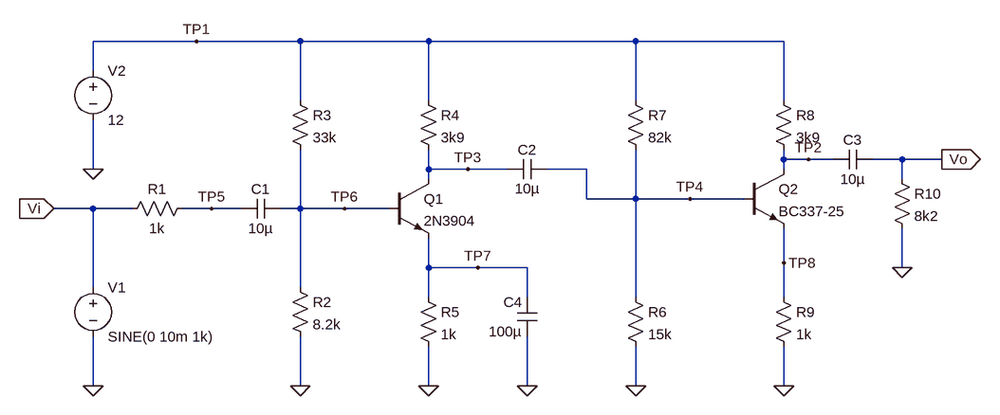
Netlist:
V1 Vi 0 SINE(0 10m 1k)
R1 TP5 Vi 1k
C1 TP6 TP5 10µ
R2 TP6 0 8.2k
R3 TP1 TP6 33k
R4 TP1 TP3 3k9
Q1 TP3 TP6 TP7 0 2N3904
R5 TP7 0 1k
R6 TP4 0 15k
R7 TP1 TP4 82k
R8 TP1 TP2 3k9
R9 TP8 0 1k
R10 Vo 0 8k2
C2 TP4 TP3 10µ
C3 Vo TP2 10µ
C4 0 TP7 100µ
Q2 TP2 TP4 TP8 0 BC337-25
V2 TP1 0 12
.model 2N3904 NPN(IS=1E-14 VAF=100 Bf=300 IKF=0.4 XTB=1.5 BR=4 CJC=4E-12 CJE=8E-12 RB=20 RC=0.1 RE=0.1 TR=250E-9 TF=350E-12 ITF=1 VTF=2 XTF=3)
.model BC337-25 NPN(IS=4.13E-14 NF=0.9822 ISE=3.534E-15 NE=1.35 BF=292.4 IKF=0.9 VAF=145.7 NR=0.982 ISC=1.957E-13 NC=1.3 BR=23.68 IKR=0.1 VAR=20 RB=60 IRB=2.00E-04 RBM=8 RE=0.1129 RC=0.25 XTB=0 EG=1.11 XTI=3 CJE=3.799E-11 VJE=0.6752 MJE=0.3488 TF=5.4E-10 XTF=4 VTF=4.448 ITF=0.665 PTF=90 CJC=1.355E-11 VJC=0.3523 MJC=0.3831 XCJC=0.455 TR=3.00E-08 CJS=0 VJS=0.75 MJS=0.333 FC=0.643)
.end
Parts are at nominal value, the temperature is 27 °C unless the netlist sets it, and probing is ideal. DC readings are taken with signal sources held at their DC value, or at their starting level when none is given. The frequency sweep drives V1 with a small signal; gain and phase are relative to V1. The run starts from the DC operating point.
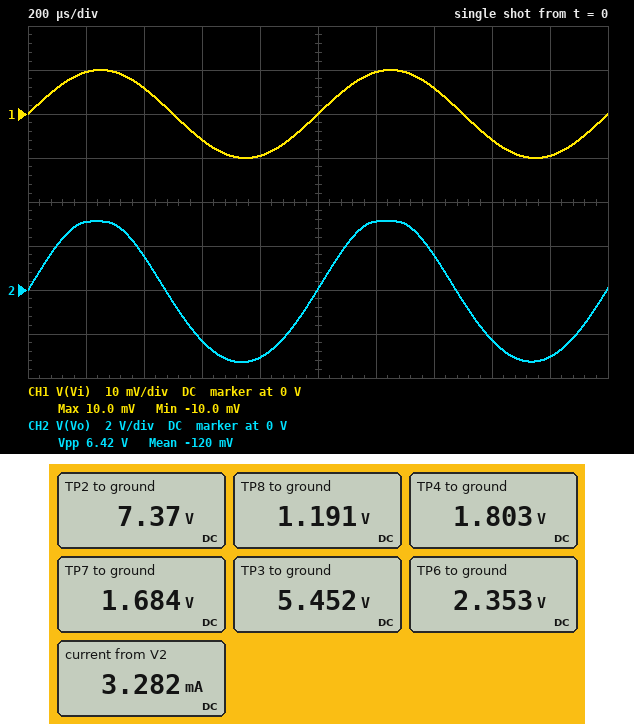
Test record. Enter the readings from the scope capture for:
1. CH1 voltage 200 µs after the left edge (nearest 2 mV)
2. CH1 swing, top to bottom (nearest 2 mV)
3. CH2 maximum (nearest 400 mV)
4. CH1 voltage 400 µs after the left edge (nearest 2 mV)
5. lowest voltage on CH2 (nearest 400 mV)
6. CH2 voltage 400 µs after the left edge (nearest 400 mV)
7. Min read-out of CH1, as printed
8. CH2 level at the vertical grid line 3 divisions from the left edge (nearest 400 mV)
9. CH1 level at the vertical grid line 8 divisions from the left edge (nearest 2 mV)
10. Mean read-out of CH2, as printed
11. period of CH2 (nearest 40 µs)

10 mV
20 mV
3.2 V
6 mV
-3.2 V
1.6 V
-10.0 mV
-2.4 V
-6 mV
-120 mV
1.00 ms
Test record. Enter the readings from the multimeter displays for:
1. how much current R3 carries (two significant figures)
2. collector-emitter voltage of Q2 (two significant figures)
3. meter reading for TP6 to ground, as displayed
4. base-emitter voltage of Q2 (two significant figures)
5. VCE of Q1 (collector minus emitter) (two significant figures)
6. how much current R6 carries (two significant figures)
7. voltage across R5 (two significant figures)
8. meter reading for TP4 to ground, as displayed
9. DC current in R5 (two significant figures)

290 µA
6.2 V
2.353 V
610 mV
3.8 V
120 µA
1.7 V
1.803 V
1.7 mA
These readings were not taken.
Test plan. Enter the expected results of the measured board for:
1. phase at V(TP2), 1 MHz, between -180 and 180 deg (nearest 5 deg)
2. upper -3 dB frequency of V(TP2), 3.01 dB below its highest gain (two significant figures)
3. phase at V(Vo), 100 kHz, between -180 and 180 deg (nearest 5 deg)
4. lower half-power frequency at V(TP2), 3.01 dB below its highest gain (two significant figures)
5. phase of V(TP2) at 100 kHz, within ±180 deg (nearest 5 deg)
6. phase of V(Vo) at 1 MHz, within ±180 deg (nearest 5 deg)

-75 deg
400 kHz
-15 deg
86 Hz
-15 deg
-75 deg
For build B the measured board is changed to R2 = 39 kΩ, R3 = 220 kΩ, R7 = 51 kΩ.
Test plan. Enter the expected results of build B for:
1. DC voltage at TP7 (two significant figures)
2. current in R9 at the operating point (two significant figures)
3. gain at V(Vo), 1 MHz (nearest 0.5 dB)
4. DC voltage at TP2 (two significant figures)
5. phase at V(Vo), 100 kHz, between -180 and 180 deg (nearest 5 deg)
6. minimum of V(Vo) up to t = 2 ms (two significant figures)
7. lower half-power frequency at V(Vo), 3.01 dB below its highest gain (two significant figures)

1.0 V
2.0 mA
41.5 dB
4.2 V
-10 deg
-1.5 V
58 Hz
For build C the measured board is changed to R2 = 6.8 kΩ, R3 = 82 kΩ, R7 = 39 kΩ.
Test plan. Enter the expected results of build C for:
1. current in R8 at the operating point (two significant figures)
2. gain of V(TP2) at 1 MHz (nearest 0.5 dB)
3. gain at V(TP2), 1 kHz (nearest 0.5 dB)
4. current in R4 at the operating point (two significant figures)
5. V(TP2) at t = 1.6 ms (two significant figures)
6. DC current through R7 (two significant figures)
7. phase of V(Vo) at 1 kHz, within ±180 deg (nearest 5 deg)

2.4 mA
14.5 dB
11.5 dB
290 µA
2.5 V
230 µA
0 deg
